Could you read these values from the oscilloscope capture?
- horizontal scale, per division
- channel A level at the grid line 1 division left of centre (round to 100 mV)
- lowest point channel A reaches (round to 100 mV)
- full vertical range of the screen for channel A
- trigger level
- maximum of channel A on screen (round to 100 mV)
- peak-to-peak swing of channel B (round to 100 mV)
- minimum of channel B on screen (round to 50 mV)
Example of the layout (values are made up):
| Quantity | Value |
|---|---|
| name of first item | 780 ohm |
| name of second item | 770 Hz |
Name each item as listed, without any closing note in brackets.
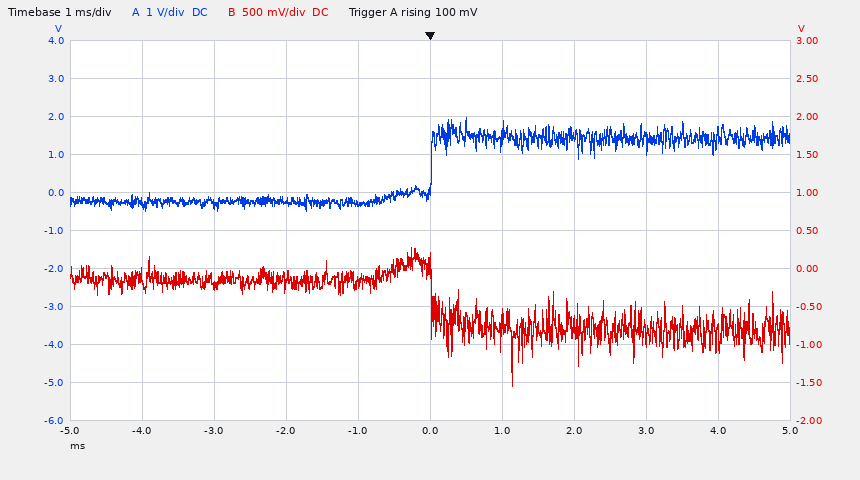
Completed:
| Quantity | Value |
|---|---|
| horizontal scale, per division | 1 ms |
| channel A level at the grid line 1 division left of centre | -300 mV |
| lowest point channel A reaches | -500 mV |
| full vertical range of the screen for channel A | 10 V |
| trigger level | 100 mV |
| maximum of channel A on screen | 2.0 V |
| peak-to-peak swing of channel B | 1.80 V |
| minimum of channel B on screen | -1.55 V |
